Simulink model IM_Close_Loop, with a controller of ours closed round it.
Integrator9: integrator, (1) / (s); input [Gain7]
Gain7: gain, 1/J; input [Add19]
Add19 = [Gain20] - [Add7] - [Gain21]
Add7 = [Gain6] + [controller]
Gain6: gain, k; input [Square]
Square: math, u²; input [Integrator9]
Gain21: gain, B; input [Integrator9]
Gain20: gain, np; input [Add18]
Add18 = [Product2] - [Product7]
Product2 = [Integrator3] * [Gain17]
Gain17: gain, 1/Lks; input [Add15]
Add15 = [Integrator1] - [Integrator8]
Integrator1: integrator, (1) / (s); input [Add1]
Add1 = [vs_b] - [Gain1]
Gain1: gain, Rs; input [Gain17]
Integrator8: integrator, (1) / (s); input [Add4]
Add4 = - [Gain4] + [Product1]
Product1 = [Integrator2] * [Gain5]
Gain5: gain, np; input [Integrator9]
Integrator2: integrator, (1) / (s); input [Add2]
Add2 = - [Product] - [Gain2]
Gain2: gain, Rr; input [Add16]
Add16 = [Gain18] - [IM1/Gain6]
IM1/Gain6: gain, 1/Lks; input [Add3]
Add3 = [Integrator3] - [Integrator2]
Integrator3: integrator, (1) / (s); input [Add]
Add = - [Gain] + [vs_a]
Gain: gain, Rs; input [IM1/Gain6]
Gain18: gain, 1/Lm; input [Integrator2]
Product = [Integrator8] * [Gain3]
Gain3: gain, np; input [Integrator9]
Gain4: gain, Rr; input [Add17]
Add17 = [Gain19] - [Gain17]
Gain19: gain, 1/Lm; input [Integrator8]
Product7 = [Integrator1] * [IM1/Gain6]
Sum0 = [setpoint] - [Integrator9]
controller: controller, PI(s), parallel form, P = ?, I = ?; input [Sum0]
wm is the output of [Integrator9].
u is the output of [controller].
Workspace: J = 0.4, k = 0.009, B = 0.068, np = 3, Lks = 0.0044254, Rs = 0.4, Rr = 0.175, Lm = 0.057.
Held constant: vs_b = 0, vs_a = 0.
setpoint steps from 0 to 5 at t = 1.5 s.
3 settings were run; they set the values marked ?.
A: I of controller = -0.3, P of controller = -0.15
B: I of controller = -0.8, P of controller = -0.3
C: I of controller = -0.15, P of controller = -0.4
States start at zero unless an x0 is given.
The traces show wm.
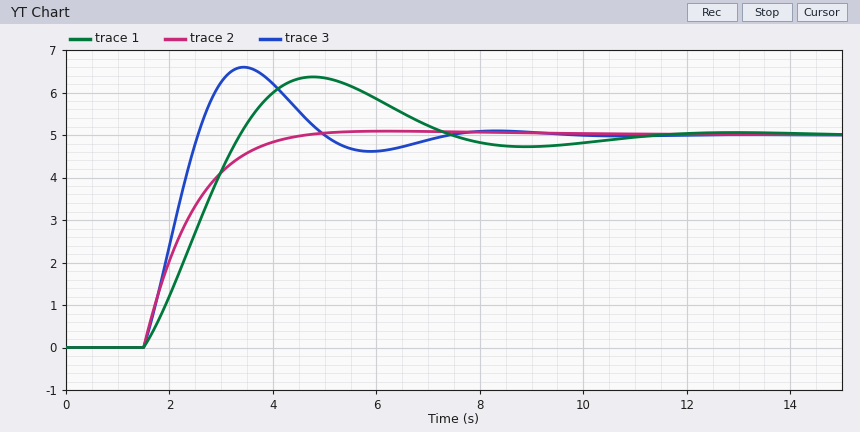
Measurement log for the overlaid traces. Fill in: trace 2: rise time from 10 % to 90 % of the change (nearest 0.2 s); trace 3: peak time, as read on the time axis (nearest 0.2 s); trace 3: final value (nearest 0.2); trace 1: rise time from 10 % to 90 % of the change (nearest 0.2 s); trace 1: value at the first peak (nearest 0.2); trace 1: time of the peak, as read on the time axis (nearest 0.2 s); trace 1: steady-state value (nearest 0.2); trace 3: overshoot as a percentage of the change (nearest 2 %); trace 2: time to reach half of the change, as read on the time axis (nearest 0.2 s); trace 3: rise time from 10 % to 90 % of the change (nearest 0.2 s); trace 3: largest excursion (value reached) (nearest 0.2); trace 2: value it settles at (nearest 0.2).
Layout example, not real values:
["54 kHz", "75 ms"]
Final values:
["1.8 s", "3.4 s", "5.0", "1.4 s", "6.4", "4.8 s", "5.0", "32 %", "2.2 s", "0.8 s", "6.6", "5.0"]
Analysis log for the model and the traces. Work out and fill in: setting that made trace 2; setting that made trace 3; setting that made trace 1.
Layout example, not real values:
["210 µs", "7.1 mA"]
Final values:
["C", "B", "A"]
